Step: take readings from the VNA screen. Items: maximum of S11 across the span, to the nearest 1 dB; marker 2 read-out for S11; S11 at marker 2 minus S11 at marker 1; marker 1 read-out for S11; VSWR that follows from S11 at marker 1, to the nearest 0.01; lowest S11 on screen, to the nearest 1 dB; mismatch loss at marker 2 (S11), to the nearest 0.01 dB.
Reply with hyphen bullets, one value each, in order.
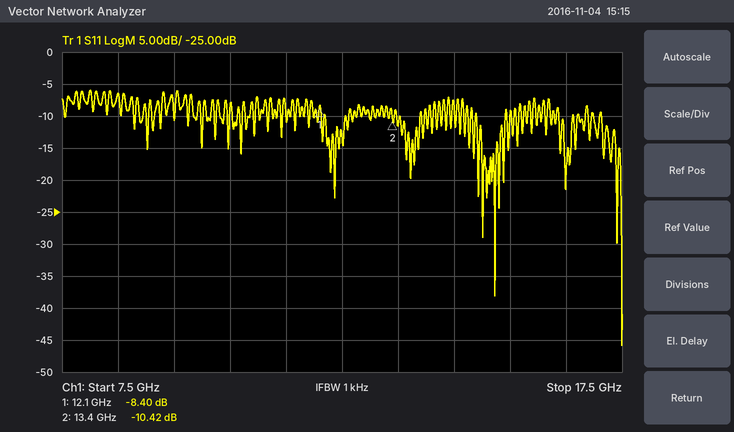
- -6 dB
- -10.42 dB
- -2.02 dB
- -8.40 dB
- 2.23
- -46 dB
- 0.41 dB
